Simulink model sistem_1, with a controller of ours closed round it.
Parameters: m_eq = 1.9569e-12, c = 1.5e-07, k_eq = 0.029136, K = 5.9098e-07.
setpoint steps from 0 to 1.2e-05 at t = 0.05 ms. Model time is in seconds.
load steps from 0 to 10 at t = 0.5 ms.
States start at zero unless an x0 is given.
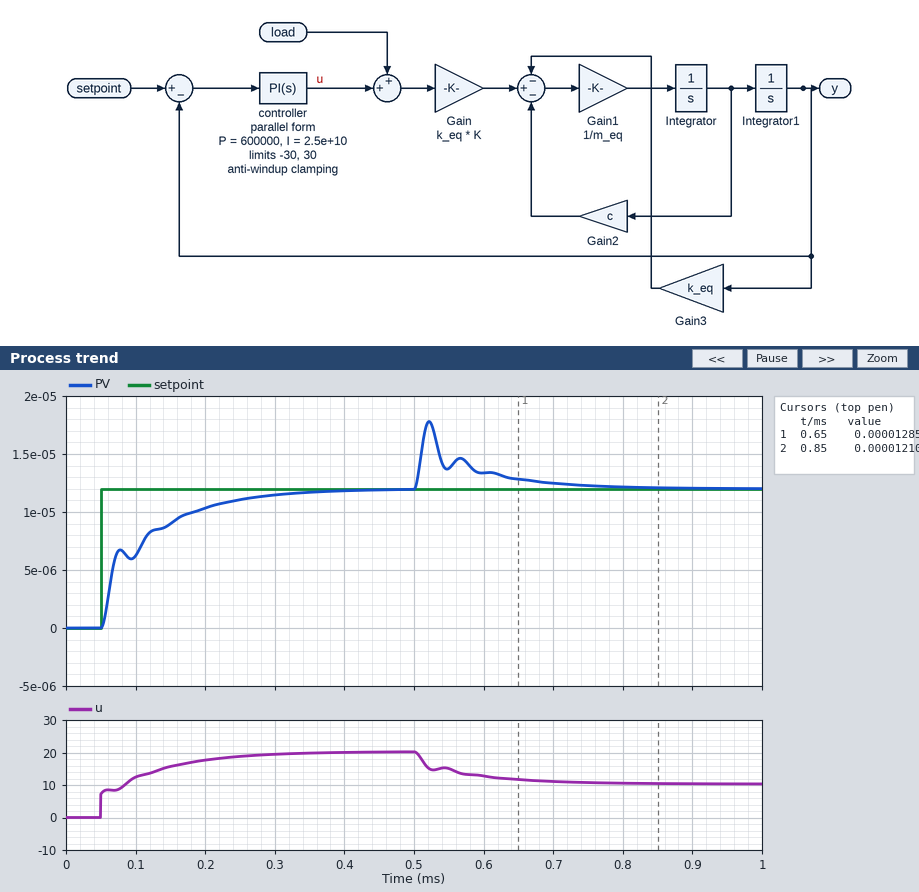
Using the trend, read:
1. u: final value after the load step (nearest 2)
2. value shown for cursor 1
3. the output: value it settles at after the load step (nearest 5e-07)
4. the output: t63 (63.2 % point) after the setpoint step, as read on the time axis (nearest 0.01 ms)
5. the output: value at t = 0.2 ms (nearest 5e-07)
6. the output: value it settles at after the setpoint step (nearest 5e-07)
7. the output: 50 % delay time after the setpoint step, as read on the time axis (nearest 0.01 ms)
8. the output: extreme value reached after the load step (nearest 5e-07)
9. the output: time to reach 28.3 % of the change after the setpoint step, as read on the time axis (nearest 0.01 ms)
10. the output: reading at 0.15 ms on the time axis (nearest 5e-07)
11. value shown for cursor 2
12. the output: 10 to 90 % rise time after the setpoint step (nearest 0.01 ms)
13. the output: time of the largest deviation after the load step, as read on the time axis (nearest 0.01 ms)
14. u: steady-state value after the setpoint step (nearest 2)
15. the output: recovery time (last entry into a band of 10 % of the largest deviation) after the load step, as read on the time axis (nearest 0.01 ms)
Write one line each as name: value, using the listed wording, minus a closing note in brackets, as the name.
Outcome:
u: final value after the load step: 10
value shown for cursor 1: 0.00001285
the output: value it settles at after the load step: 0.0000120
the output: t63 (63.2 % point) after the setpoint step, as read on the time axis: 0.11 ms
the output: value at t = 0.2 ms: 0.0000105
the output: value it settles at after the setpoint step: 0.0000120
the output: 50 % delay time after the setpoint step, as read on the time axis: 0.07 ms
the output: extreme value reached after the load step: 0.0000180
the output: time to reach 28.3 % of the change after the setpoint step, as read on the time axis: 0.06 ms
the output: reading at 0.15 ms on the time axis: 0.0000090
value shown for cursor 2: 0.00001210
the output: 10 to 90 % rise time after the setpoint step: 0.17 ms
the output: time of the largest deviation after the load step, as read on the time axis: 0.52 ms
u: steady-state value after the setpoint step: 20
the output: recovery time (last entry into a band of 10 % of the largest deviation) after the load step, as read on the time axis: 0.68 ms
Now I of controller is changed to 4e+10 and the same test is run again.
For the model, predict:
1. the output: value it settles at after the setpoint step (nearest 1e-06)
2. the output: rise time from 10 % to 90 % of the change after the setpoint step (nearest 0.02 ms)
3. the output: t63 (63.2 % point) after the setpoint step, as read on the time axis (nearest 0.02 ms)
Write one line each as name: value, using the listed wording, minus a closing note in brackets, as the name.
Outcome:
the output: value it settles at after the setpoint step: 0.000012
the output: rise time from 10 % to 90 % of the change after the setpoint step: 0.10 ms
the output: t63 (63.2 % point) after the setpoint step, as read on the time axis: 0.08 ms
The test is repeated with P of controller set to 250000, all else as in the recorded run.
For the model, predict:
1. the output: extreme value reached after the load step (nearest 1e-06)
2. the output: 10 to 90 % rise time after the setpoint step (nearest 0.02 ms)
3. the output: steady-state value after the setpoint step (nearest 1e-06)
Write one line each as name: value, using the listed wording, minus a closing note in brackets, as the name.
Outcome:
the output: extreme value reached after the load step: 0.000019
the output: 10 to 90 % rise time after the setpoint step: 0.16 ms
the output: steady-state value after the setpoint step: 0.000012
